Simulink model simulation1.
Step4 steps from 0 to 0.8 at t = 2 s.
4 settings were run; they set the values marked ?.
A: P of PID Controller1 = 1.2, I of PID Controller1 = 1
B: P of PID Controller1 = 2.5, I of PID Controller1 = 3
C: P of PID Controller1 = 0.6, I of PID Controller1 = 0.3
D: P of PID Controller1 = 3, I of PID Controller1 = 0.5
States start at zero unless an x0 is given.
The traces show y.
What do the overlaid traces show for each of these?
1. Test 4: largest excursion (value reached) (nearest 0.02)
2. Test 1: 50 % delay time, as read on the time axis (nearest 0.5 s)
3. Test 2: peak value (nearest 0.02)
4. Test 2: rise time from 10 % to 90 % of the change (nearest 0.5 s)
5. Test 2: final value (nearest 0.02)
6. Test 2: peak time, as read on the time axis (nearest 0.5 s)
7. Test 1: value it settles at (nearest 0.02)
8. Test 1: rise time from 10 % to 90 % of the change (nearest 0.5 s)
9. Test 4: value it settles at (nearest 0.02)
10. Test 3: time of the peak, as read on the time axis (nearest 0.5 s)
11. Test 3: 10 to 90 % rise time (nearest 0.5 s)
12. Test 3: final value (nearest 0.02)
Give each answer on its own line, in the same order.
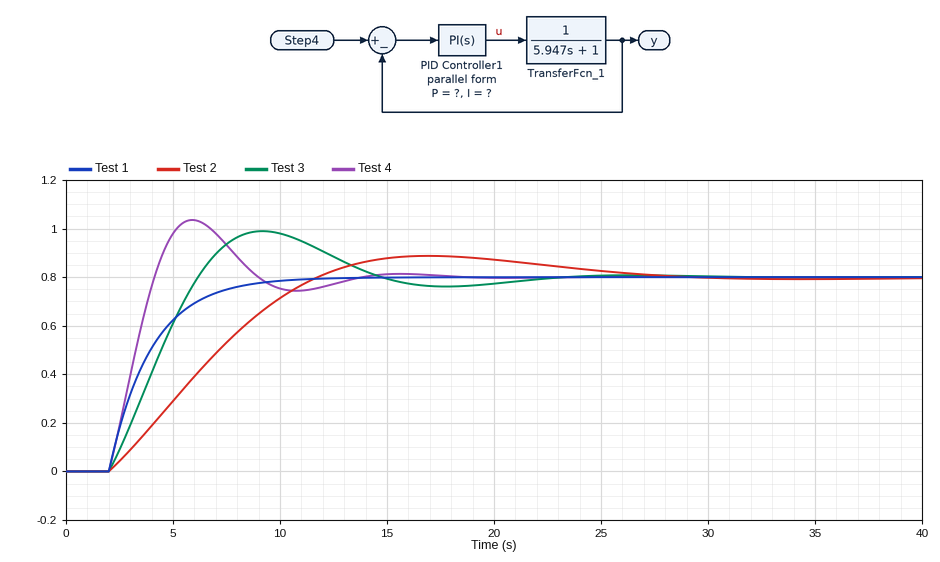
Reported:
1.04
3.5 s
0.88
7.0 s
0.80
17.0 s
0.80
4.5 s
0.80
9.0 s
3.0 s
0.80
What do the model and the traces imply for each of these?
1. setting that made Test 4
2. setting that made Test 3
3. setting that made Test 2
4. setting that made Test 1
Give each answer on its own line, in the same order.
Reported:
B
A
C
D
